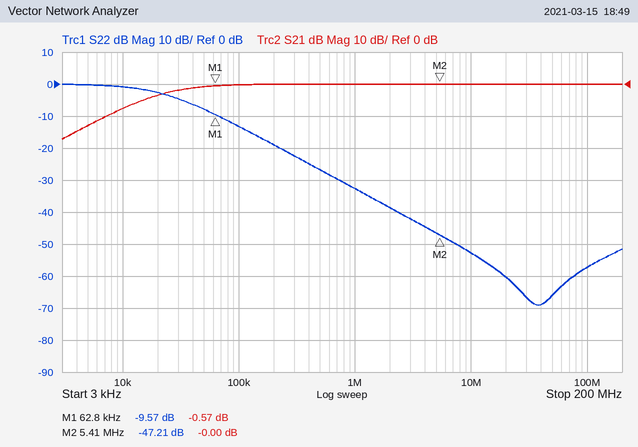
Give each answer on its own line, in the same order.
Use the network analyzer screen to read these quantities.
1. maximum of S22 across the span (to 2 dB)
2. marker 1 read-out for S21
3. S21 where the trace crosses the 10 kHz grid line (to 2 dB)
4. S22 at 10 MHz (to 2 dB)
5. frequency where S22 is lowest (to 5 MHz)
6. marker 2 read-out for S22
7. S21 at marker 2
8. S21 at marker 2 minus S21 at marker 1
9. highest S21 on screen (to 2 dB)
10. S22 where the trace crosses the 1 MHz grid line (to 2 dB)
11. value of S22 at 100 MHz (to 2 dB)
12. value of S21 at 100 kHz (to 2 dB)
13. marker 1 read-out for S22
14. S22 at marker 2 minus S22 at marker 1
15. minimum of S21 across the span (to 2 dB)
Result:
0 dB
-0.57 dB
-8 dB
-52 dB
40 MHz
-47.21 dB
-0.00 dB
0.57 dB
0 dB
-32 dB
-58 dB
0 dB
-9.57 dB
-37.64 dB
-18 dB
